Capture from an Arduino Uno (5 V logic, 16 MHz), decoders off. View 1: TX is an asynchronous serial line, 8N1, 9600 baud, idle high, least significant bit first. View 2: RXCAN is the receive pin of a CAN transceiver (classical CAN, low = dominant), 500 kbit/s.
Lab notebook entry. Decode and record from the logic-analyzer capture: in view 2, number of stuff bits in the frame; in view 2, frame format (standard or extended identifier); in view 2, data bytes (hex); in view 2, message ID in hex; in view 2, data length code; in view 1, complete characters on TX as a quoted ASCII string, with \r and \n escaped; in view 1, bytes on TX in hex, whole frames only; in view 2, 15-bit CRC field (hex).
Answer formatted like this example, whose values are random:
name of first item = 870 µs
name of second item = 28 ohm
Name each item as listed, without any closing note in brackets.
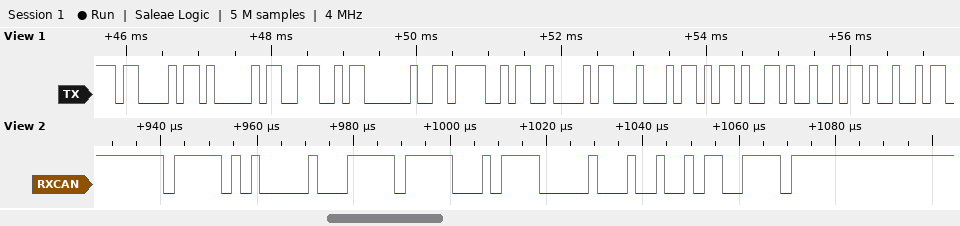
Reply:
in view 2, number of stuff bits in the frame = 5
in view 2, frame format = standard
in view 2, data bytes = FF 2F 00
in view 2, message ID in hex = 0x7E8
in view 2, data length code = 3
in view 1, complete characters on TX as a quoted ASCII string, with \r and \n escaped = "CAN OBD-II"
in view 1, bytes on TX in hex, whole frames only = 43 41 4E 20 4F 42 44 2D 49 49
in view 2, 15-bit CRC field = 0x4967
